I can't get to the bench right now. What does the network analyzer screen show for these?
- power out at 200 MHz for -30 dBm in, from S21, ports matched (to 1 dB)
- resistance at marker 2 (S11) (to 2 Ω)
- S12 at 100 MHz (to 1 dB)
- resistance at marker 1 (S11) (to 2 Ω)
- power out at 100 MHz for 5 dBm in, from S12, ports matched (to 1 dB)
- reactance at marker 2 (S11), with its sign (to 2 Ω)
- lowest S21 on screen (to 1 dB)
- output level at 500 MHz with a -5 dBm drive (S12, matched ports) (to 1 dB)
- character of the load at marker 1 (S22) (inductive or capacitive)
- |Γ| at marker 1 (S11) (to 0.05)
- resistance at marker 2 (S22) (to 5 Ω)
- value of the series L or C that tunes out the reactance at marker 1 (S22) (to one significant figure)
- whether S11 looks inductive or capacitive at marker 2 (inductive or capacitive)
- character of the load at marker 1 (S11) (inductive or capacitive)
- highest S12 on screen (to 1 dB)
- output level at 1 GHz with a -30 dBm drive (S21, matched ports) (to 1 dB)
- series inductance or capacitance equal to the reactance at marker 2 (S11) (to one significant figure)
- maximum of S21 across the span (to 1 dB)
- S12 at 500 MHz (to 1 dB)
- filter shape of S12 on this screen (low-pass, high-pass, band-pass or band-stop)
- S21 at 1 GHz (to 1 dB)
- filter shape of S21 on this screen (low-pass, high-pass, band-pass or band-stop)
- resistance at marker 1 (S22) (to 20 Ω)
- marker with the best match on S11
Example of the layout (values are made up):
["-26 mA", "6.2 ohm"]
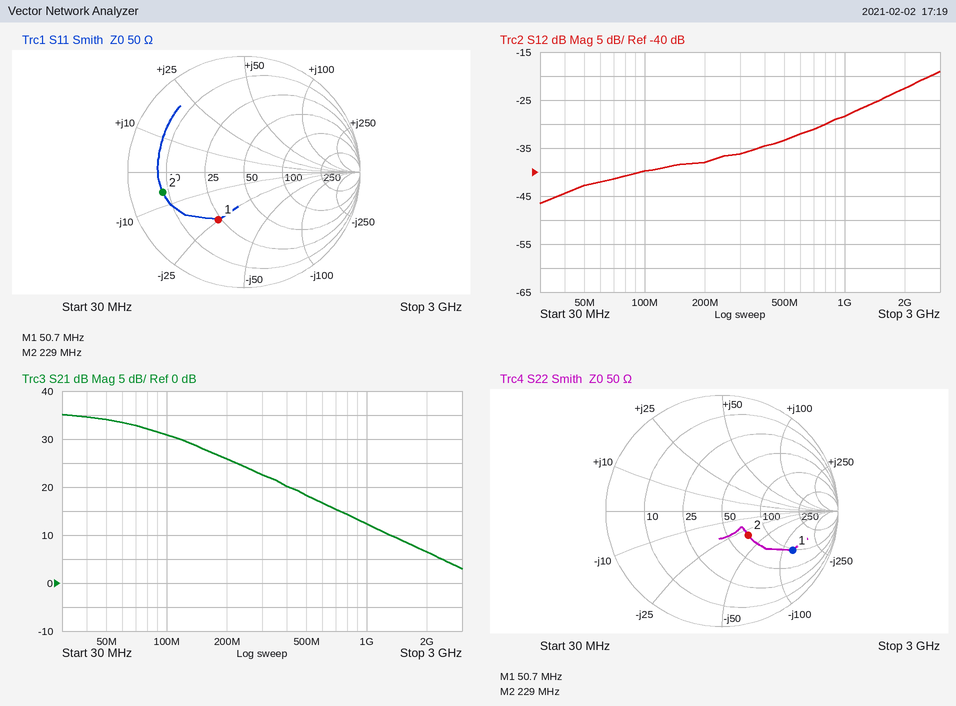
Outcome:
["-4 dBm", "8 Ω", "-40 dB", "24 Ω", "-35 dBm", "-6 Ω", "3 dB", "-38 dBm", "capacitive", "0.45", "70 Ω", "400 nH", "capacitive", "capacitive", "-19 dB", "-18 dBm", "100 pF", "35 dB", "-33 dB", "high-pass", "12 dB", "low-pass", "100 Ω", "marker 1"]
